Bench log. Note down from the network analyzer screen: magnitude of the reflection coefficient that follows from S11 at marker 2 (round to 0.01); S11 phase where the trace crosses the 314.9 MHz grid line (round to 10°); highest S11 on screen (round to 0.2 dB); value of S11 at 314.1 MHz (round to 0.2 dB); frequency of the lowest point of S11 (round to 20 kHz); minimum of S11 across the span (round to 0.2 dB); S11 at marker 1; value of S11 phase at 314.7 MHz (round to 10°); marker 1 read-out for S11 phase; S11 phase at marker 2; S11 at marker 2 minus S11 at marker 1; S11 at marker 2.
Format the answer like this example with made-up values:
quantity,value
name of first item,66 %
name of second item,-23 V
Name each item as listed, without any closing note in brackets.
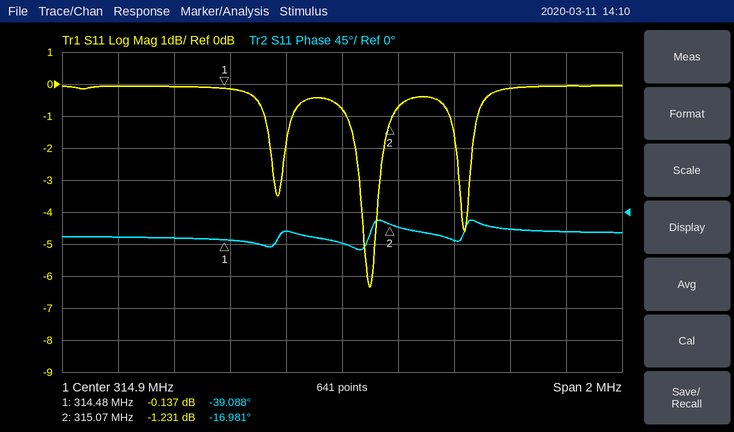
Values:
quantity,value
magnitude of the reflection coefficient that follows from S11 at marker 2,0.87
S11 phase where the trace crosses the 314.9 MHz grid line,-40°
highest S11 on screen,0.0 dB
value of S11 at 314.1 MHz,0.0 dB
frequency of the lowest point of S11,315.00 MHz
minimum of S11 across the span,-6.4 dB
S11 at marker 1,-0.137 dB
value of S11 phase at 314.7 MHz,-30°
marker 1 read-out for S11 phase,-39.088°
S11 phase at marker 2,-16.981°
S11 at marker 2 minus S11 at marker 1,-1.094 dB
S11 at marker 2,-1.231 dB
